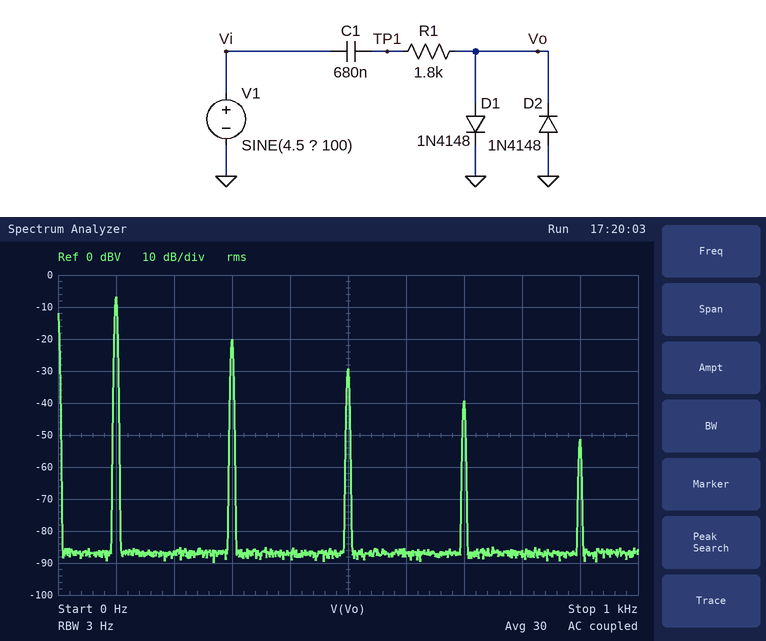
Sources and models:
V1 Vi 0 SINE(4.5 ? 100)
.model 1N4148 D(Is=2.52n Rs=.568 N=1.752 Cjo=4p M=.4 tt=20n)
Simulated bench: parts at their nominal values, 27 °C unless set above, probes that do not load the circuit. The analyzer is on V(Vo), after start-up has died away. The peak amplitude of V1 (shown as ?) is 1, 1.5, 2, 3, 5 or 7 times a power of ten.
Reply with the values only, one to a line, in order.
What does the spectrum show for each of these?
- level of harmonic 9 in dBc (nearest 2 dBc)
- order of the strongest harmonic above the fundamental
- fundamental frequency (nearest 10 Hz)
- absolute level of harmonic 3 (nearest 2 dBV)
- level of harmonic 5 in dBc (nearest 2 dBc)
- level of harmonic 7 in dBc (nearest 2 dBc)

-44 dBc
3
100 Hz
-20 dBV
-22 dBc
-32 dBc
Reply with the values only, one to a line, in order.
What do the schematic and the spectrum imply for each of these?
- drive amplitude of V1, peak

1.5 V
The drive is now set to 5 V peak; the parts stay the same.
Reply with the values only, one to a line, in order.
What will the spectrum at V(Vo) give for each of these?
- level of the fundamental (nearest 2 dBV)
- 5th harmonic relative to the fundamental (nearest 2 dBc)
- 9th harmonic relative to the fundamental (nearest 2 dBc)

-6 dBV
-16 dBc
-24 dBc
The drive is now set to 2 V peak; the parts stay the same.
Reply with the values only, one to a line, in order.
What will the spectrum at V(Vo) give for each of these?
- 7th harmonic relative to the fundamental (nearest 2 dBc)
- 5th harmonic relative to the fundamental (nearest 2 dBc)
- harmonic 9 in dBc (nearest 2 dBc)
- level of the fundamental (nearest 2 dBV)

-28 dBc
-20 dBc
-36 dBc
-6 dBV
